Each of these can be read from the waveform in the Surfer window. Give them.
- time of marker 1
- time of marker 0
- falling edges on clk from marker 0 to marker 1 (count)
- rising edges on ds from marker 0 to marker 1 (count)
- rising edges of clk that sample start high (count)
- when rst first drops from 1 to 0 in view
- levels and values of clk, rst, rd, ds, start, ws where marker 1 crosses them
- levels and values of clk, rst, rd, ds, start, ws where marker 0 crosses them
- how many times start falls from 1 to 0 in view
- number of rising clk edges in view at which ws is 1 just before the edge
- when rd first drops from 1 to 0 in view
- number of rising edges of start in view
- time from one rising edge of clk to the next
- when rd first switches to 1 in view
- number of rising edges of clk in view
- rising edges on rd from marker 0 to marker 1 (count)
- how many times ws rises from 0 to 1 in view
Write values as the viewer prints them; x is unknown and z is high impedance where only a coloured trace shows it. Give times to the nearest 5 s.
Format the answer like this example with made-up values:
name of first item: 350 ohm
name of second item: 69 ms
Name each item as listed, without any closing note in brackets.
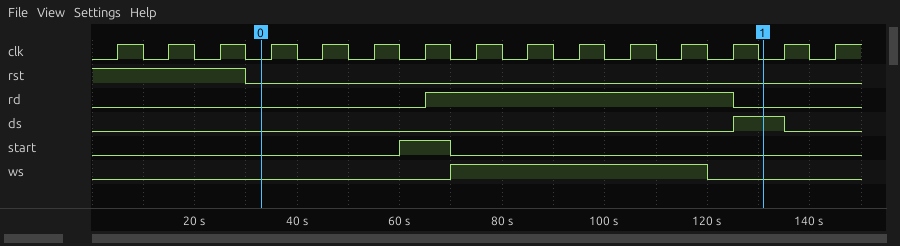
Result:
time of marker 1: 130 s
time of marker 0: 35 s
falling edges on clk from marker 0 to marker 1: 10
rising edges on ds from marker 0 to marker 1: 1
rising edges of clk that sample start high: 1
when rst first drops from 1 to 0 in view: 30 s
levels and values of clk, rst, rd, ds, start, ws where marker 1 crosses them: clk=0, rst=0, rd=0, ds=1, start=0, ws=0
levels and values of clk, rst, rd, ds, start, ws where marker 0 crosses them: clk=0, rst=0, rd=0, ds=0, start=0, ws=0
how many times start falls from 1 to 0 in view: 1
number of rising clk edges in view at which ws is 1 just before the edge: 5
when rd first drops from 1 to 0 in view: 125 s
number of rising edges of start in view: 1
time from one rising edge of clk to the next: 10 s
when rd first switches to 1 in view: 65 s
number of rising edges of clk in view: 15
rising edges on rd from marker 0 to marker 1: 1
how many times ws rises from 0 to 1 in view: 1
